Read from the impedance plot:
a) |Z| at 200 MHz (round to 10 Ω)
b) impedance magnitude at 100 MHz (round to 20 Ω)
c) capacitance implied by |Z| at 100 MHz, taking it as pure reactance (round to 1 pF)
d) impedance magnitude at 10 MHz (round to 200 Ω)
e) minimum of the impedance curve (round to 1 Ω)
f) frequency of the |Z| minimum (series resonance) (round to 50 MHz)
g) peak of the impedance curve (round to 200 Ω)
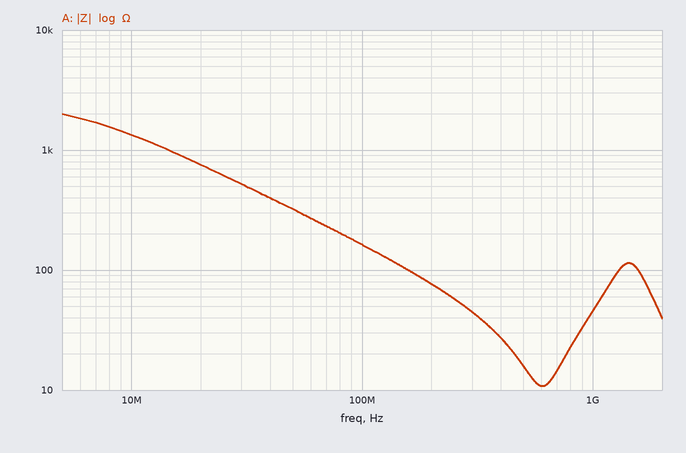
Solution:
80 Ω
160 Ω
10 pF
1.4 kΩ
11 Ω
600 MHz
2.0 kΩ
